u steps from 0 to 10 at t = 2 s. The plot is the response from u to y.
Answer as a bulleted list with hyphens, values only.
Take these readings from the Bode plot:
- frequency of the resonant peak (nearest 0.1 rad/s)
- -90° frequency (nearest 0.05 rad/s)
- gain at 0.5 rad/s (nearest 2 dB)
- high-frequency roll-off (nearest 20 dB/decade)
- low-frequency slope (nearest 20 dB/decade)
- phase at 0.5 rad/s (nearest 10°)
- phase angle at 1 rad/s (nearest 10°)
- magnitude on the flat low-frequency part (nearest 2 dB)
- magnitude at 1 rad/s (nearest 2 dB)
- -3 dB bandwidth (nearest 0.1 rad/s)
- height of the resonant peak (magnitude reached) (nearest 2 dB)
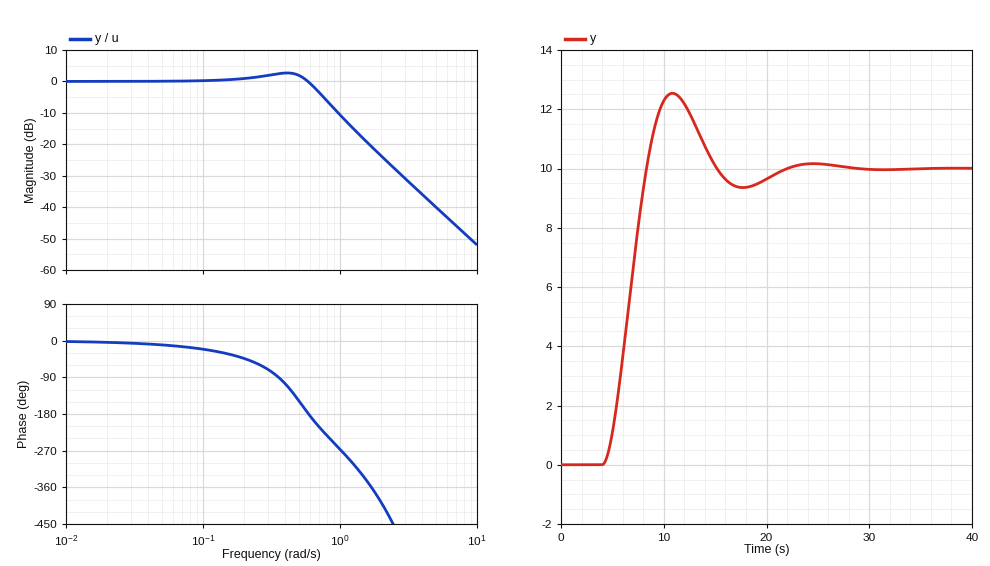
- 0.4 rad/s
- 0.35 rad/s
- 2 dB
- -40 dB/decade
- 0 dB/decade
- -150°
- -270°
- 0 dB
- -10 dB
- 0.7 rad/s
- 2 dB
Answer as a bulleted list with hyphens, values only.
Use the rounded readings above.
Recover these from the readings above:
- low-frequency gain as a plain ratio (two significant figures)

- 1.0
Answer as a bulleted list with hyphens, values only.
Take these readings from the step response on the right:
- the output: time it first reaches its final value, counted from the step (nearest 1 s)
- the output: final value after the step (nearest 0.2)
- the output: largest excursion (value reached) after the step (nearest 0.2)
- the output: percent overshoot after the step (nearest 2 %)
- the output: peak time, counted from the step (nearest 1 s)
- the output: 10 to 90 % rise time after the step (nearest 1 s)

- 6 s
- 10.0
- 12.6
- 26 %
- 9 s
- 3 s
